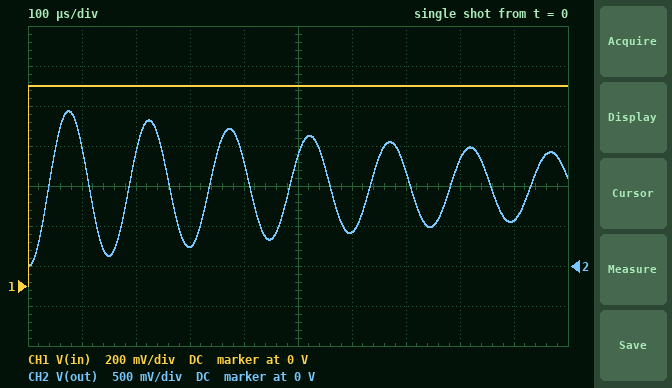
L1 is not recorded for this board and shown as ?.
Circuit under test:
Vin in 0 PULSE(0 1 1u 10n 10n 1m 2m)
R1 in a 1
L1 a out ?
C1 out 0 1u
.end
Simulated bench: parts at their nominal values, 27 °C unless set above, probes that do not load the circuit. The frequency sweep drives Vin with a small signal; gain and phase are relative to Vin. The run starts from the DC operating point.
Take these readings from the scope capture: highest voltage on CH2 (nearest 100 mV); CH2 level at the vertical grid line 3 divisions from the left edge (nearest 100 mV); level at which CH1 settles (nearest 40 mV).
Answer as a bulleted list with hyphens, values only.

- 1.9 V
- 200 mV
- 1.00 V
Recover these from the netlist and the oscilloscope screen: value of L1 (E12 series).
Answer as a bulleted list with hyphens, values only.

- 560 µH
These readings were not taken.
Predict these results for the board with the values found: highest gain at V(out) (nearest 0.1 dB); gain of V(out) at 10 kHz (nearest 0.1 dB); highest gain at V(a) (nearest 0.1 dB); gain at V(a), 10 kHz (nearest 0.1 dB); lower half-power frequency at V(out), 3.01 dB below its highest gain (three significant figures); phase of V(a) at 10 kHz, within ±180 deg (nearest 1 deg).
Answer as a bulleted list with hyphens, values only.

- 27.5 dB
- -1.7 dB
- 0 dB
- 0 dB
- 6.58 kHz
- 3 deg
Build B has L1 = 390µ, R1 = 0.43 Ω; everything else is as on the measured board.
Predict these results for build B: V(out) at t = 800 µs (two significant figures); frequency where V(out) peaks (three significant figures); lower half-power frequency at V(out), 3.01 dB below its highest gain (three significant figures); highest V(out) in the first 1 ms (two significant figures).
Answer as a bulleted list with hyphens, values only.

- 1.6 V
- 8.06 kHz
- 7.97 kHz
- 2.0 V
